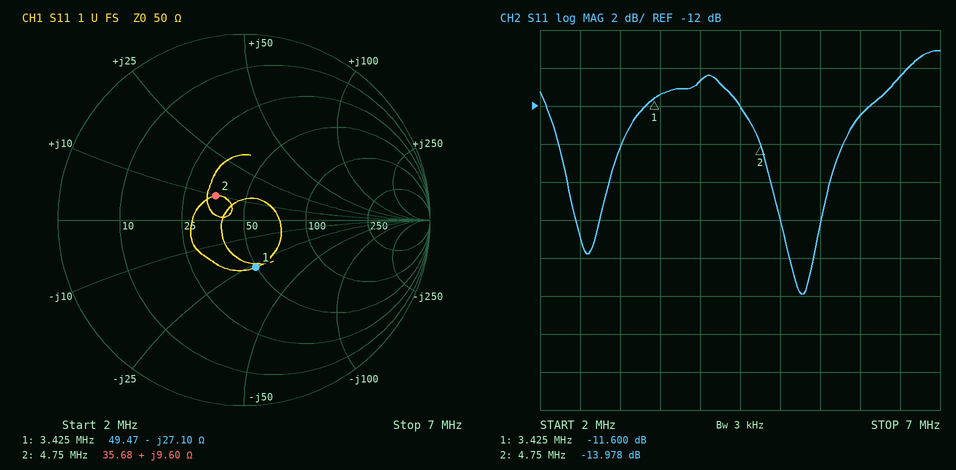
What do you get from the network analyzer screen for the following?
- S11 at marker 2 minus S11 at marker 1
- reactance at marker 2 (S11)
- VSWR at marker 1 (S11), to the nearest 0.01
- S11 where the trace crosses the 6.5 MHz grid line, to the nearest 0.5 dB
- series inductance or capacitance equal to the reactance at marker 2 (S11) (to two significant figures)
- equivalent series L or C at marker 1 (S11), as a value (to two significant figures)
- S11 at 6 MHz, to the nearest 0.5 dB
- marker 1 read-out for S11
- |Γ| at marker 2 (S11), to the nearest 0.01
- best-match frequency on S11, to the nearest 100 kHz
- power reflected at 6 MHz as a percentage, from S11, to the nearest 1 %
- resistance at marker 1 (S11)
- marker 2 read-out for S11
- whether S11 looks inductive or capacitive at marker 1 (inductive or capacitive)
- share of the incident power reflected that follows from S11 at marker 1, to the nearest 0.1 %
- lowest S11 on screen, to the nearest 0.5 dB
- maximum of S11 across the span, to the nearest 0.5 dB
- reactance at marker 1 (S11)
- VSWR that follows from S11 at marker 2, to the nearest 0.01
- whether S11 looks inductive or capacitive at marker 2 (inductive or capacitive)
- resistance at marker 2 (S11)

-2.378 dB
+9.60 Ω
1.71
-10.5 dB
320 nH
1.7 nF
-12.5 dB
-11.600 dB
0.20
5.3 MHz
6 %
49.47 Ω
-13.978 dB
capacitive
6.9 %
-22.0 dB
-9.0 dB
-27.10 Ω
1.50
inductive
35.68 Ω
